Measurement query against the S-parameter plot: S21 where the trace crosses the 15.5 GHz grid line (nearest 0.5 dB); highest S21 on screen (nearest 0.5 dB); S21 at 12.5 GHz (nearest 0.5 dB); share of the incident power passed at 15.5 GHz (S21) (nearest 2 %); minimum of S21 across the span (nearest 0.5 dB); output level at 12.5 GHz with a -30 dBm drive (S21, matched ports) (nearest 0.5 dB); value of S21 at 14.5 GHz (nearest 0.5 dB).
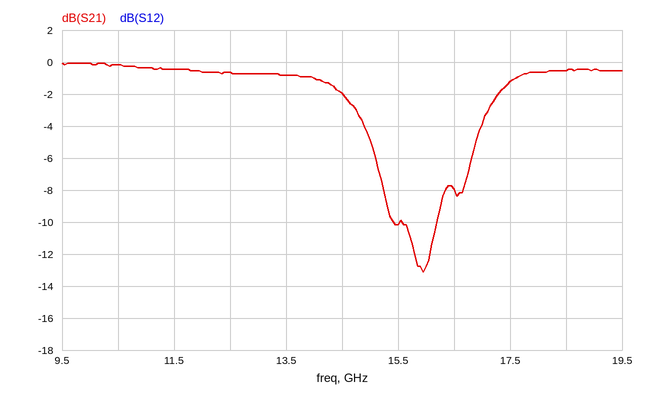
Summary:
-10.0 dB
0.0 dB
-0.5 dB
10 %
-13.0 dB
-30.5 dBm
-2.0 dB
